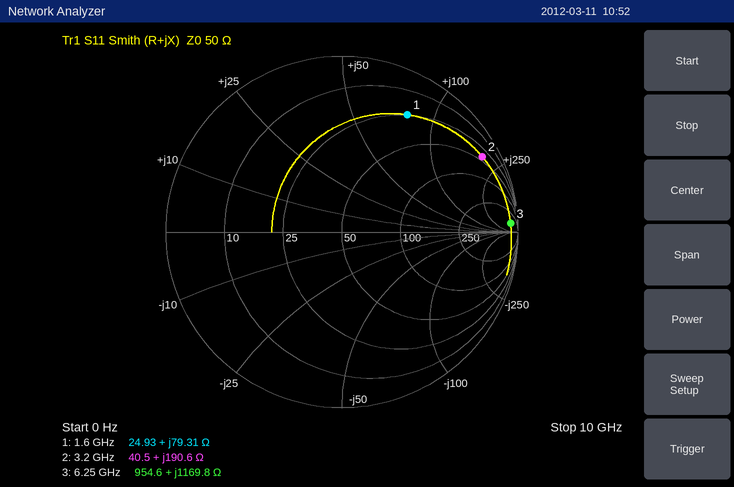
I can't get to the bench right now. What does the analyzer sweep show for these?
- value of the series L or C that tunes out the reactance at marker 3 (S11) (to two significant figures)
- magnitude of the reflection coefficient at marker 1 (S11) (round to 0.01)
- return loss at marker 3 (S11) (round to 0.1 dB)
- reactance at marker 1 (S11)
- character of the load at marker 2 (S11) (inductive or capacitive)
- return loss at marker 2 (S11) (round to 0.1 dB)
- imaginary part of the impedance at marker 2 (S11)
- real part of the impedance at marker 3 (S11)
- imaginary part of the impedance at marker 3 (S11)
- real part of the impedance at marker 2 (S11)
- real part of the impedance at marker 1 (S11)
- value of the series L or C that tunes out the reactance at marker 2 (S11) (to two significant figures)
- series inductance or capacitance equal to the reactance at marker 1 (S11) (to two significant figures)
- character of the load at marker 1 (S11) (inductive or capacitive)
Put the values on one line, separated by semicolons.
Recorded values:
22 fF; 0.76; 0.4 dB; +79.31 Ω; inductive; 0.9 dB; +190.6 Ω; 954.6 Ω; +1169.8 Ω; 40.5 Ω; 24.93 Ω; 260 fF; 7.9 nH; inductive
